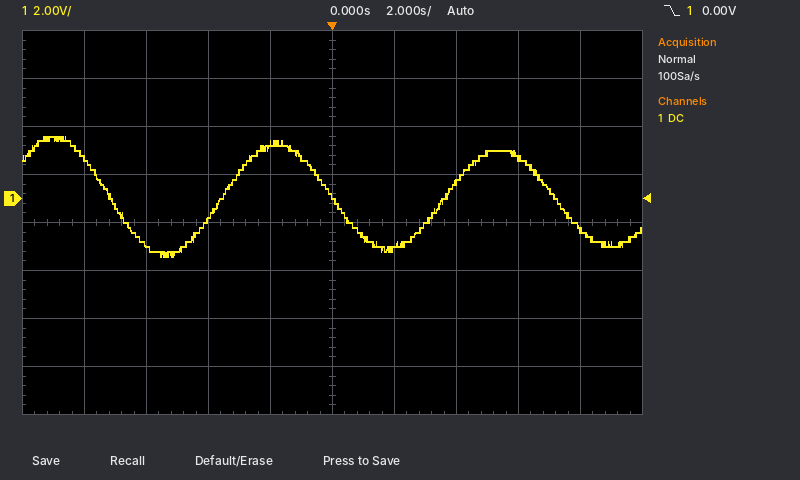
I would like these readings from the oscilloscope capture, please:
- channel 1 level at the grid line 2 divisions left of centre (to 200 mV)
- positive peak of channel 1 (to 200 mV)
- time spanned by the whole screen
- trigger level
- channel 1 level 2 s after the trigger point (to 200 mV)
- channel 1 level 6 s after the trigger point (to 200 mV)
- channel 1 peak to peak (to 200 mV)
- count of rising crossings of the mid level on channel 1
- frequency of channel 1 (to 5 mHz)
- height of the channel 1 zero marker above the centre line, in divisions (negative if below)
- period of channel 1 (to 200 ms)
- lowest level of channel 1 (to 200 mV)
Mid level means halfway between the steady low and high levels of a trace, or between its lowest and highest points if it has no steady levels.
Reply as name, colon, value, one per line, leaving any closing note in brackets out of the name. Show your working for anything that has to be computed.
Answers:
channel 1 level at the grid line 2 divisions left of centre: -800 mV
positive peak of channel 1: 2.6 V
time spanned by the whole screen: 20 s
trigger level: 0.00 V
channel 1 level 2 s after the trigger point: -2.0 V
channel 1 level 6 s after the trigger point: 1.8 V
channel 1 peak to peak: 2.6 V − (-2.4 V) = 5.0 V
count of rising crossings of the mid level on channel 1: 2
frequency of channel 1: 1 / 7.2 s ≈ 139 mHz, so 140 mHz to the nearest 5 mHz
height of the channel 1 zero marker above the centre line, in divisions: +0.5 div
period of channel 1: 7.2 s
lowest level of channel 1: -2.4 V
